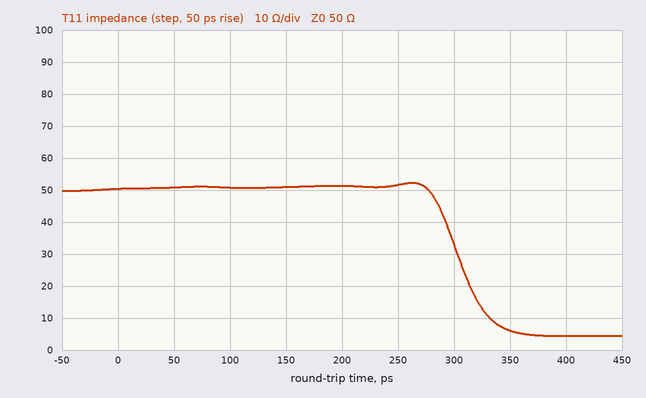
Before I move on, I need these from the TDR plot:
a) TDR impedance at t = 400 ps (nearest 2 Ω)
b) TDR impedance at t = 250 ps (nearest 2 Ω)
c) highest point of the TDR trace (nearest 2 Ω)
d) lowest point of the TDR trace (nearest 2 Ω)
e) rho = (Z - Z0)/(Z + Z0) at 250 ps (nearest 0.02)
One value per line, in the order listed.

4 Ω
52 Ω
52 Ω
4 Ω
+0.02
